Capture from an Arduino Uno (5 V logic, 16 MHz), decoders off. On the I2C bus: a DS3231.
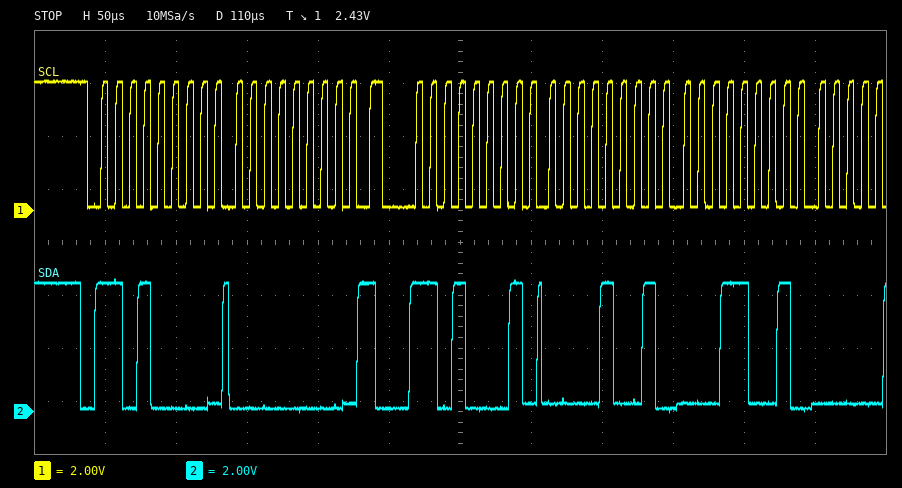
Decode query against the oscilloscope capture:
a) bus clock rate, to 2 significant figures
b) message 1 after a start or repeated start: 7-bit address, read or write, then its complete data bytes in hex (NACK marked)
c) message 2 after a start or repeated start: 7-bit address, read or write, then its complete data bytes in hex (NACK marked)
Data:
100 kHz
0x68 write: 00
0x68 read: 09 19
